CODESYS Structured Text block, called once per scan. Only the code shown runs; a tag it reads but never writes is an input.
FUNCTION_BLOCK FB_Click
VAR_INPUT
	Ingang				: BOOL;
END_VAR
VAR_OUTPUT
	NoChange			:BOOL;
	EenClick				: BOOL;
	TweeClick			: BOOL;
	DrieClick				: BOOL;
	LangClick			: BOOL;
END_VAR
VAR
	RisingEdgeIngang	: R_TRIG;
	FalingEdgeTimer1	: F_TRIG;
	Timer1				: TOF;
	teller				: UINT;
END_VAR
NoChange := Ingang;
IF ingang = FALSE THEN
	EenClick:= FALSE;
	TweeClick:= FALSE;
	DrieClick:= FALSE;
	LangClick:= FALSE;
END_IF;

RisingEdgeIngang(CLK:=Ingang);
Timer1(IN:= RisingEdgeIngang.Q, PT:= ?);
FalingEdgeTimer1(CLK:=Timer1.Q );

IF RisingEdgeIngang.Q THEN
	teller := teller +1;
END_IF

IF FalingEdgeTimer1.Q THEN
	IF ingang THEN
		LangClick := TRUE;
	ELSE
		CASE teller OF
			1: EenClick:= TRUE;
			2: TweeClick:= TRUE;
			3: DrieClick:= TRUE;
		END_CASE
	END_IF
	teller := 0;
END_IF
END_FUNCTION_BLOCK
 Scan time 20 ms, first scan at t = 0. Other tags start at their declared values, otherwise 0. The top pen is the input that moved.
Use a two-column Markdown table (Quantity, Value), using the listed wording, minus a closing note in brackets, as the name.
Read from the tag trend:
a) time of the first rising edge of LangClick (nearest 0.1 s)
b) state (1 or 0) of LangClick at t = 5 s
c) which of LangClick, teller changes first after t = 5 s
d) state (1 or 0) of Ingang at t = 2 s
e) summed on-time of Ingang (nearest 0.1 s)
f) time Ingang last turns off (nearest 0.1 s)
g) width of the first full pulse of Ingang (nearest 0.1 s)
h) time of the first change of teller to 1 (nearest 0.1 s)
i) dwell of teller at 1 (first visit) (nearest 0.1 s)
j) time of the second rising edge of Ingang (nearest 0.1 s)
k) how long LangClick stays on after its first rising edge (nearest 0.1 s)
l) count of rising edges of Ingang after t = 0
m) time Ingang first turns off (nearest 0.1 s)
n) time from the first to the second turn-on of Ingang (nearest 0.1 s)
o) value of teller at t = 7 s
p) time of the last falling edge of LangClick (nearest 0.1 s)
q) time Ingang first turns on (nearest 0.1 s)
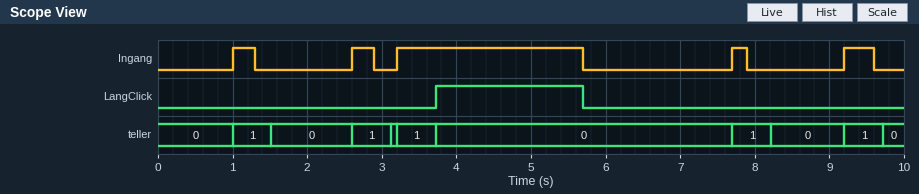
| Quantity | Value |
|---|---|
| time of the first rising edge of LangClick | 3.7 s |
| state (1 or 0) of LangClick at t = 5 s | 1 |
| which of LangClick, teller changes first after t = 5 s | LangClick |
| state (1 or 0) of Ingang at t = 2 s | 0 |
| summed on-time of Ingang | 3.7 s |
| time Ingang last turns off | 9.6 s |
| width of the first full pulse of Ingang | 0.3 s |
| time of the first change of teller to 1 | 1.0 s |
| dwell of teller at 1 (first visit) | 0.5 s |
| time of the second rising edge of Ingang | 2.6 s |
| how long LangClick stays on after its first rising edge | 2.0 s |
| count of rising edges of Ingang after t = 0 | 5 |
| time Ingang first turns off | 1.3 s |
| time from the first to the second turn-on of Ingang | 1.6 s |
| value of teller at t = 7 s | 0 |
| time of the last falling edge of LangClick | 5.7 s |
| time Ingang first turns on | 1.0 s |
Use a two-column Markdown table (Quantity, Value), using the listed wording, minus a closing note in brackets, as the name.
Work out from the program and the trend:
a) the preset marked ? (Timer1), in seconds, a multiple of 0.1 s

| Quantity | Value |
|---|---|
| the preset marked ? (Timer1), in seconds, a multiple of 0.1 s | 0.5 s |
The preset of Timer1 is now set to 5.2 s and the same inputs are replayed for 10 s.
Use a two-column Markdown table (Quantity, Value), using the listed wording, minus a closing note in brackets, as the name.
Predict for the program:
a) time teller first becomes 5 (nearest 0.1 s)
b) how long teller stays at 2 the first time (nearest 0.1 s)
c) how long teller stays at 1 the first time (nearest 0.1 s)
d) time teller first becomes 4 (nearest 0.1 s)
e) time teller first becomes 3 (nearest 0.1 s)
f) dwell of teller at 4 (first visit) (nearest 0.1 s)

| Quantity | Value |
|---|---|
| time teller first becomes 5 | 9.2 s |
| how long teller stays at 2 the first time | 0.6 s |
| how long teller stays at 1 the first time | 1.6 s |
| time teller first becomes 4 | 7.7 s |
| time teller first becomes 3 | 3.2 s |
| dwell of teller at 4 (first visit) | 1.5 s |
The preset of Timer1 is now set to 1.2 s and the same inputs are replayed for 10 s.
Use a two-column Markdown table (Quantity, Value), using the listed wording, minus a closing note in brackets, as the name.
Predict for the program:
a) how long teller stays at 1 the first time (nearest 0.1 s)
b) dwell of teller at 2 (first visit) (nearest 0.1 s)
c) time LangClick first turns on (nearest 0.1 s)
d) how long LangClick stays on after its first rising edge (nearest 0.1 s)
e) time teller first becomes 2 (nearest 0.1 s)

| Quantity | Value |
|---|---|
| how long teller stays at 1 the first time | 1.2 s |
| dwell of teller at 2 (first visit) | 1.2 s |
| time LangClick first turns on | 4.4 s |
| how long LangClick stays on after its first rising edge | 1.3 s |
| time teller first becomes 2 | 3.2 s |
